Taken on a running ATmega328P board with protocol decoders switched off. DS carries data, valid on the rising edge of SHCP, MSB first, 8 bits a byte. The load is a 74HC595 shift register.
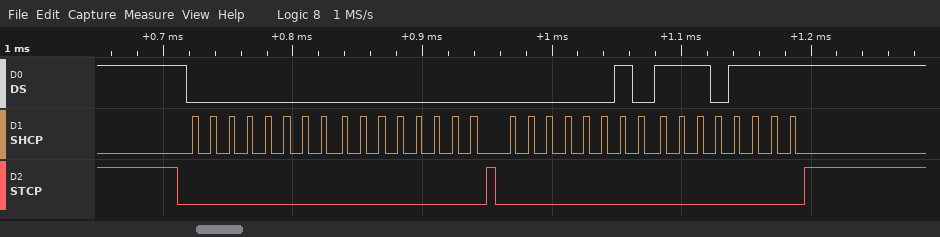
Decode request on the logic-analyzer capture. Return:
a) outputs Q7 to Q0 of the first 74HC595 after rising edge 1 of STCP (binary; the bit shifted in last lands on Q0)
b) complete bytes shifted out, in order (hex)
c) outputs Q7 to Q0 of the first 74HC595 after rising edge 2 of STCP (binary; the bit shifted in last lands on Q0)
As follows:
00000000
00 00 02 EF
11101111
